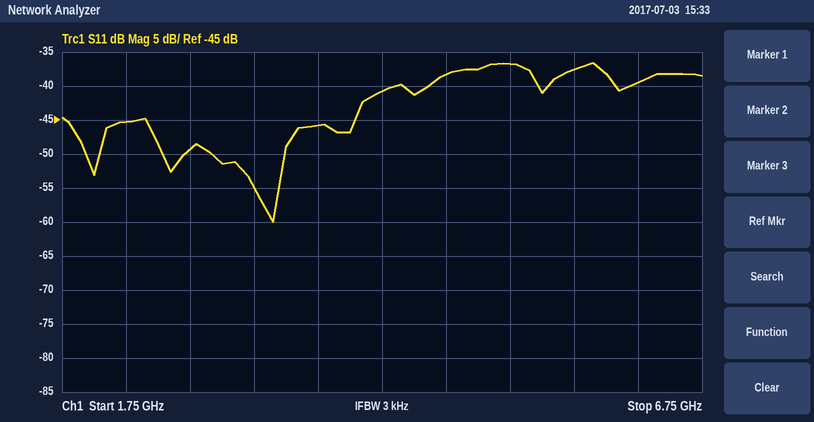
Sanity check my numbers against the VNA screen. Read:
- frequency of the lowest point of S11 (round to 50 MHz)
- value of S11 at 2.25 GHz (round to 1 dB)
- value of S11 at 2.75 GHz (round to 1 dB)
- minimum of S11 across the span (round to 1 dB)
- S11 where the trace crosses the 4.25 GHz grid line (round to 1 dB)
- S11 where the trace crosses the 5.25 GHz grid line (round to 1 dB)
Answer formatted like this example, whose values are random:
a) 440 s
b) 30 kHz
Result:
a) 3.40 GHz
b) -45 dB
c) -49 dB
d) -60 dB
e) -41 dB
f) -37 dB
